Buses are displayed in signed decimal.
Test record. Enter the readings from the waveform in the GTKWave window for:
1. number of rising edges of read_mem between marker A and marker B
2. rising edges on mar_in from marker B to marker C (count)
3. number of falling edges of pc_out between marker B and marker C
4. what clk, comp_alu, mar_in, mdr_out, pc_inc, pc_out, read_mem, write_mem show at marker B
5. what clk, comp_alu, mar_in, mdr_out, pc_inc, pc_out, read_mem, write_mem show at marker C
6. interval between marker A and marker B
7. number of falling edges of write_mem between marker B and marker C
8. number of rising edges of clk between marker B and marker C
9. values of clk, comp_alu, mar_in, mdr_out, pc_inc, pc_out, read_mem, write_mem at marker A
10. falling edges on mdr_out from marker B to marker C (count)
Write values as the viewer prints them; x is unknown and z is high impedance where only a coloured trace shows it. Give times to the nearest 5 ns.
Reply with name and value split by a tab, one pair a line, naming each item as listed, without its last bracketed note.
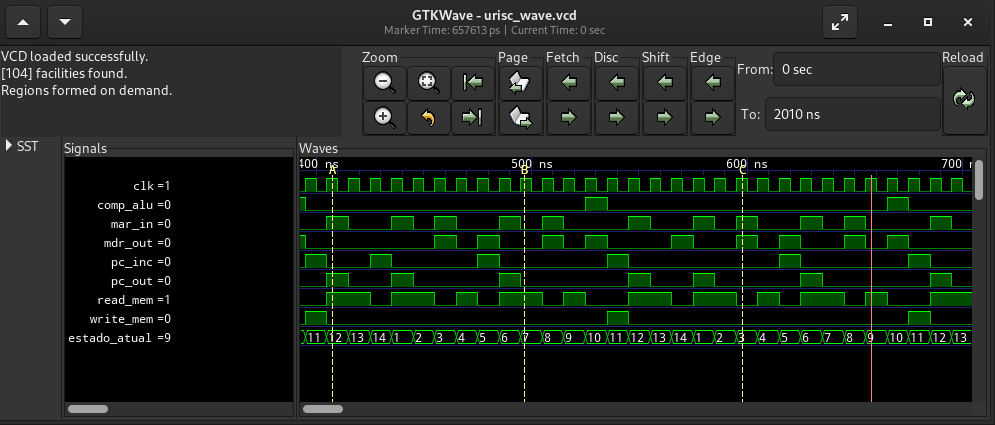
number of rising edges of read_mem between marker A and marker B	3
rising edges on mar_in from marker B to marker C	4
number of falling edges of pc_out between marker B and marker C	2
what clk, comp_alu, mar_in, mdr_out, pc_inc, pc_out, read_mem, write_mem show at marker B	clk=1, comp_alu=0, mar_in=0, mdr_out=0, pc_inc=0, pc_out=0, read_mem=1, write_mem=0
what clk, comp_alu, mar_in, mdr_out, pc_inc, pc_out, read_mem, write_mem show at marker C	clk=1, comp_alu=0, mar_in=1, mdr_out=1, pc_inc=0, pc_out=0, read_mem=0, write_mem=0
interval between marker A and marker B	90 ns
number of falling edges of write_mem between marker B and marker C	1
number of rising edges of clk between marker B and marker C	10
values of clk, comp_alu, mar_in, mdr_out, pc_inc, pc_out, read_mem, write_mem at marker A	clk=1, comp_alu=0, mar_in=1, mdr_out=0, pc_inc=0, pc_out=1, read_mem=1, write_mem=0
falling edges on mdr_out from marker B to marker C	3
